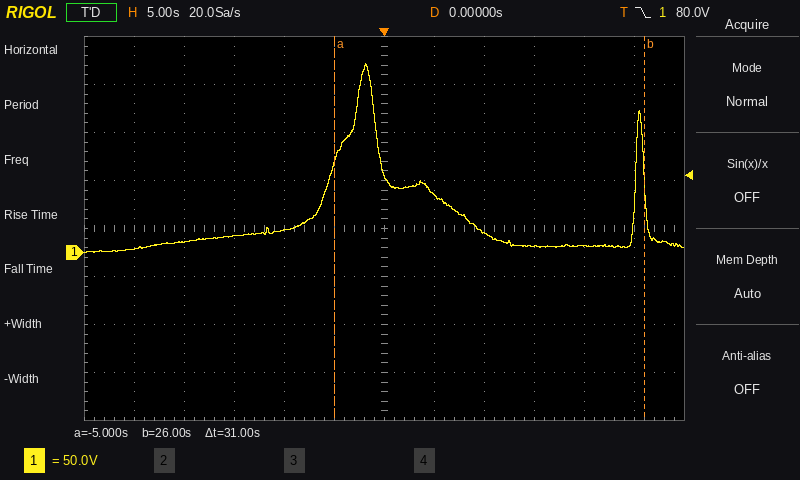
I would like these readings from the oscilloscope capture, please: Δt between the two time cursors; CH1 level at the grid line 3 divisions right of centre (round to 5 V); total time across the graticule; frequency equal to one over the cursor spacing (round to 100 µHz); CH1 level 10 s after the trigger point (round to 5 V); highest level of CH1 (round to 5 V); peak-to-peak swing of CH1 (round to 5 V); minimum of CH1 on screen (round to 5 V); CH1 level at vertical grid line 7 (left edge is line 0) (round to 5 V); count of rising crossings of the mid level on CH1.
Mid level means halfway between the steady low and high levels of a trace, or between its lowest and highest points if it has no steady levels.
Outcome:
31 s
5 V
60 s
32.3 mHz
20 V
195 V
195 V
0 V
60 V
2
